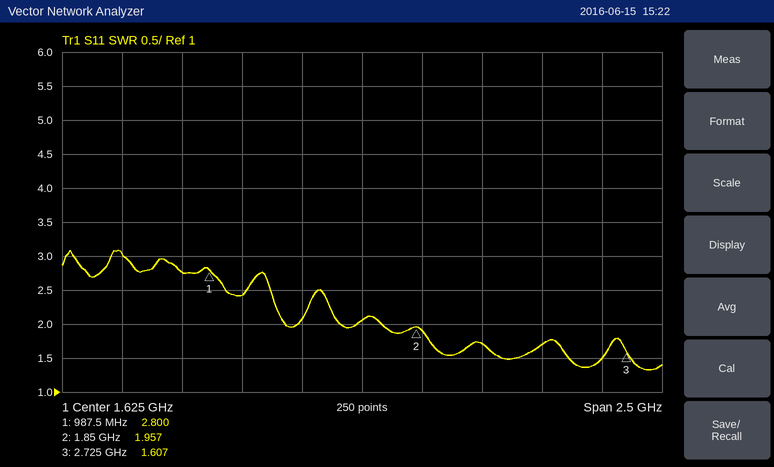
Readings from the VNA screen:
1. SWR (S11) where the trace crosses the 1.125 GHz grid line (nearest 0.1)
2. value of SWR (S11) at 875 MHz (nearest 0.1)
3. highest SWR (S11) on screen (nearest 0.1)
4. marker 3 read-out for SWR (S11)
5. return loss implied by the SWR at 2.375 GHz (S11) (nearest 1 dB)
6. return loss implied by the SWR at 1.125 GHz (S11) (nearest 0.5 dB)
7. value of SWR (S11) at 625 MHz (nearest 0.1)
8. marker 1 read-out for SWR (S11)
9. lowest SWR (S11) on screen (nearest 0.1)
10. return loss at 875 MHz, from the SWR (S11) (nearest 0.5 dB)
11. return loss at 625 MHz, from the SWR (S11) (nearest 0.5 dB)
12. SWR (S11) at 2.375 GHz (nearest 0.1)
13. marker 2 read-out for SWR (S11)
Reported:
2.4
2.8
3.1
1.607
12 dB
7.5 dB
3.0
2.800
1.3
6.5 dB
6.0 dB
1.7
1.957
